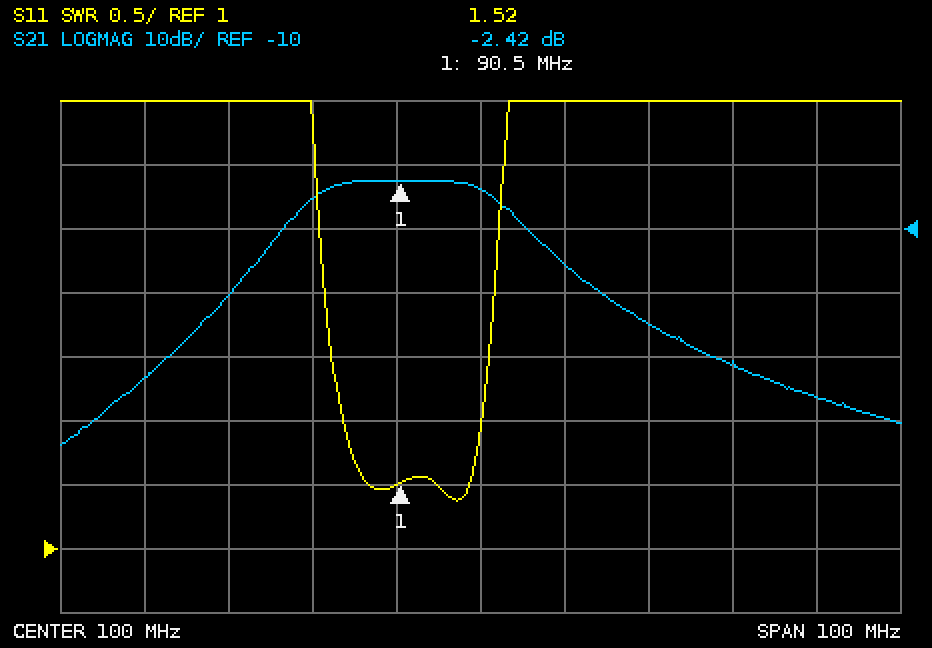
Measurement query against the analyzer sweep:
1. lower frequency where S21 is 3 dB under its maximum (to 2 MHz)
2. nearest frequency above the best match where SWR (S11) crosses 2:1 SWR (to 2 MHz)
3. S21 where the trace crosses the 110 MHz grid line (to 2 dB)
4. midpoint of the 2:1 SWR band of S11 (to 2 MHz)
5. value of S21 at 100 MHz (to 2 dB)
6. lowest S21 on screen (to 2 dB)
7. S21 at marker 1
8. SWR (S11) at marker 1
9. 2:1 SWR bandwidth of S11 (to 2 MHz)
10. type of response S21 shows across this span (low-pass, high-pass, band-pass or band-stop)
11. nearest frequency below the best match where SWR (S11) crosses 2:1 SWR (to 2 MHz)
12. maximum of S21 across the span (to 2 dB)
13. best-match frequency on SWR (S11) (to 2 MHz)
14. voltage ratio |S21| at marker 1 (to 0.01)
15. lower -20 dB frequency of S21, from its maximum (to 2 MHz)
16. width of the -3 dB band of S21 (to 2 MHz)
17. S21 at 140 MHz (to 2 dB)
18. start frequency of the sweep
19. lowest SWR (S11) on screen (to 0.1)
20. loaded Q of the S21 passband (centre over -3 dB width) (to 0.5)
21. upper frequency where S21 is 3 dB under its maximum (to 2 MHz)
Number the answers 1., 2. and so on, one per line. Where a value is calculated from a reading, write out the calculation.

1. 80 MHz
2. 100 MHz
3. -16 dB
4. 92 MHz
5. -4 dB
6. -44 dB
7. -2.42 dB
8. 1.52
9. 100 MHz − 84 MHz = 16 MHz
10. band-pass
11. 84 MHz
12. -2 dB
13. 98 MHz
14. 10^(-2.42/20) ≈ 0.76
15. 68 MHz
16. 102 MHz − 80 MHz = 22 MHz
17. -36 dB
18. 50 MHz
19. 1.4
20. 91 MHz / 22 MHz ≈ 4.14, so 4.0 to the nearest 0.5
21. 102 MHz
